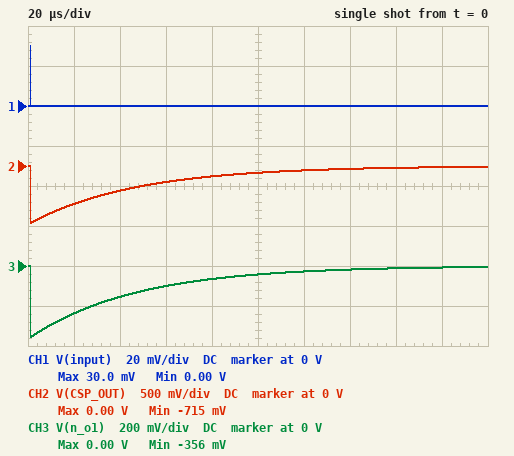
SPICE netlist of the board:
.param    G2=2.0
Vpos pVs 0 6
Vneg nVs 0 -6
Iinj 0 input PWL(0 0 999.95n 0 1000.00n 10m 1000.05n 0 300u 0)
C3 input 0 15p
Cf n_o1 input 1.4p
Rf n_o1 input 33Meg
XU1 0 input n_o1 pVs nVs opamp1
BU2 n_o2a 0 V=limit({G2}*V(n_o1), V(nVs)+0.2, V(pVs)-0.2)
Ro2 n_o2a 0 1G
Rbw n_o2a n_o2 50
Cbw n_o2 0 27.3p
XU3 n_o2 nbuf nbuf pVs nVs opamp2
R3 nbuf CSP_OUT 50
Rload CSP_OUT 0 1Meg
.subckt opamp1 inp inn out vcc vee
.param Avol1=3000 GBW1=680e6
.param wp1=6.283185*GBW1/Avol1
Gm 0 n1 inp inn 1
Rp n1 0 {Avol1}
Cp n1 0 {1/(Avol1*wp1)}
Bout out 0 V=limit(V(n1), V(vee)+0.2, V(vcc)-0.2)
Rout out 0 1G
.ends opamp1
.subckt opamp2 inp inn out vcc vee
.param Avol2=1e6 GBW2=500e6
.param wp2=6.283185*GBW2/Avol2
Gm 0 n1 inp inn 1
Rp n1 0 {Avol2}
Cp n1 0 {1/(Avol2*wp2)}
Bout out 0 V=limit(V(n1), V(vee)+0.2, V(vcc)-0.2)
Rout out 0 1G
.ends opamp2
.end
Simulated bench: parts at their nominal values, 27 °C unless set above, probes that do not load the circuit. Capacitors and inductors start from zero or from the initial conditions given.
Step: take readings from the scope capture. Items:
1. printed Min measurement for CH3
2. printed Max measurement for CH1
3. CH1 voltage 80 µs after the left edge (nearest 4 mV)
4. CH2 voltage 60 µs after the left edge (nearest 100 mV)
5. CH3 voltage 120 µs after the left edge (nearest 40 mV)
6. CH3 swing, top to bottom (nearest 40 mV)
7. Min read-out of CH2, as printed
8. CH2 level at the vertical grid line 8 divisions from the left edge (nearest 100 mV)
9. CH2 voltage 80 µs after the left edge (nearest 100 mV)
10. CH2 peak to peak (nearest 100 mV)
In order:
-356 mV
30.0 mV
0 V
-200 mV
-40 mV
360 mV
-715 mV
0 V
-100 mV
700 mV
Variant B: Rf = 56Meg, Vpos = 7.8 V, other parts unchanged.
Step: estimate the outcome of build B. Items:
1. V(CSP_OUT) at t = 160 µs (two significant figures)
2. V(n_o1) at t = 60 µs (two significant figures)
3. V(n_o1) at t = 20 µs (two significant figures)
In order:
-95 mV
-170 mV
-280 mV
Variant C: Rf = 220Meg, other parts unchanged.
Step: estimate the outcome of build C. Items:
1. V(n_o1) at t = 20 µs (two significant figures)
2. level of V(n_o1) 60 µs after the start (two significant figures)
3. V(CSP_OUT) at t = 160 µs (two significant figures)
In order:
-340 mV
-300 mV
-430 mV
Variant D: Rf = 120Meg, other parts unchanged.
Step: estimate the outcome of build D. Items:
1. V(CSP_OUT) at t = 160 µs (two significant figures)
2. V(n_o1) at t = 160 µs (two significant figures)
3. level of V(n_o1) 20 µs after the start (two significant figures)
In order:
-280 mV
-140 mV
-320 mV
